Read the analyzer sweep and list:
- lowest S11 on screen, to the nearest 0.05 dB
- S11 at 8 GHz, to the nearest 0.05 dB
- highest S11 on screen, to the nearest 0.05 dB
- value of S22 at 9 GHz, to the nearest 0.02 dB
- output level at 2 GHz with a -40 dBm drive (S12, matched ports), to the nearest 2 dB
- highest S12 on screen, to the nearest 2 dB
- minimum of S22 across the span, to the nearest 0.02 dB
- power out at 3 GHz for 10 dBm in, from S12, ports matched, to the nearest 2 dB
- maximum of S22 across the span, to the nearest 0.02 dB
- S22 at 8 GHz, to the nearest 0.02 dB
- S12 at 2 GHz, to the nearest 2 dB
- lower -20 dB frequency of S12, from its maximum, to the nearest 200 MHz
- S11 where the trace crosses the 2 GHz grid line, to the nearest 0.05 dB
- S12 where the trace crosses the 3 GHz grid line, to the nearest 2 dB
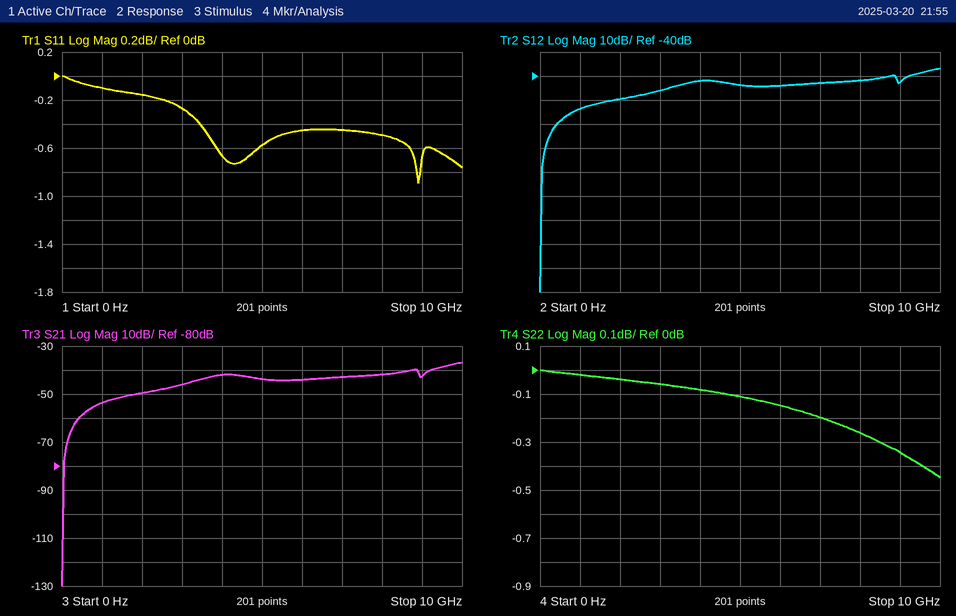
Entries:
-0.90 dB
-0.50 dB
0.00 dB
-0.34 dB
-90 dBm
-36 dB
-0.44 dB
-36 dBm
0.00 dB
-0.26 dB
-50 dB
600 MHz
-0.15 dB
-46 dB
